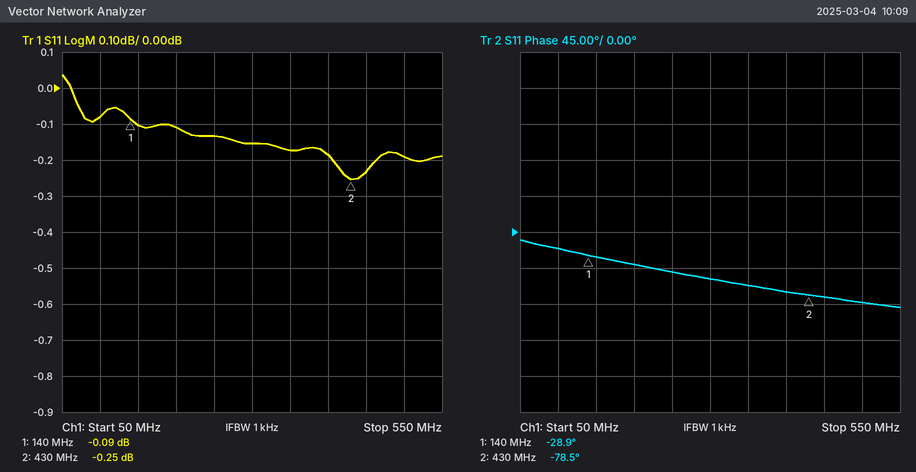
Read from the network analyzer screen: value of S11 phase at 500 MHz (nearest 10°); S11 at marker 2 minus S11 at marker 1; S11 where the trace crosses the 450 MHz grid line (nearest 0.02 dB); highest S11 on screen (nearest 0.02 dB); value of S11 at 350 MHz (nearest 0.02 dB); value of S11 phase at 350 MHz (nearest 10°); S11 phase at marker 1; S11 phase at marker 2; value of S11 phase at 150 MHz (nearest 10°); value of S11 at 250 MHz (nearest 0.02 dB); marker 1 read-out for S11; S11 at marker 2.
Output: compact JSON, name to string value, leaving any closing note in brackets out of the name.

{"value of S11 phase at 500 MHz": "-90°", "S11 at marker 2 minus S11 at marker 1": "-0.16 dB", "S11 where the trace crosses the 450 MHz grid line": "-0.24 dB", "highest S11 on screen": "0.04 dB", "value of S11 at 350 MHz": "-0.18 dB", "value of S11 phase at 350 MHz": "-70°", "S11 phase at marker 1": "-28.9°", "S11 phase at marker 2": "-78.5°", "value of S11 phase at 150 MHz": "-30°", "value of S11 at 250 MHz": "-0.14 dB", "marker 1 read-out for S11": "-0.09 dB", "S11 at marker 2": "-0.25 dB"}
